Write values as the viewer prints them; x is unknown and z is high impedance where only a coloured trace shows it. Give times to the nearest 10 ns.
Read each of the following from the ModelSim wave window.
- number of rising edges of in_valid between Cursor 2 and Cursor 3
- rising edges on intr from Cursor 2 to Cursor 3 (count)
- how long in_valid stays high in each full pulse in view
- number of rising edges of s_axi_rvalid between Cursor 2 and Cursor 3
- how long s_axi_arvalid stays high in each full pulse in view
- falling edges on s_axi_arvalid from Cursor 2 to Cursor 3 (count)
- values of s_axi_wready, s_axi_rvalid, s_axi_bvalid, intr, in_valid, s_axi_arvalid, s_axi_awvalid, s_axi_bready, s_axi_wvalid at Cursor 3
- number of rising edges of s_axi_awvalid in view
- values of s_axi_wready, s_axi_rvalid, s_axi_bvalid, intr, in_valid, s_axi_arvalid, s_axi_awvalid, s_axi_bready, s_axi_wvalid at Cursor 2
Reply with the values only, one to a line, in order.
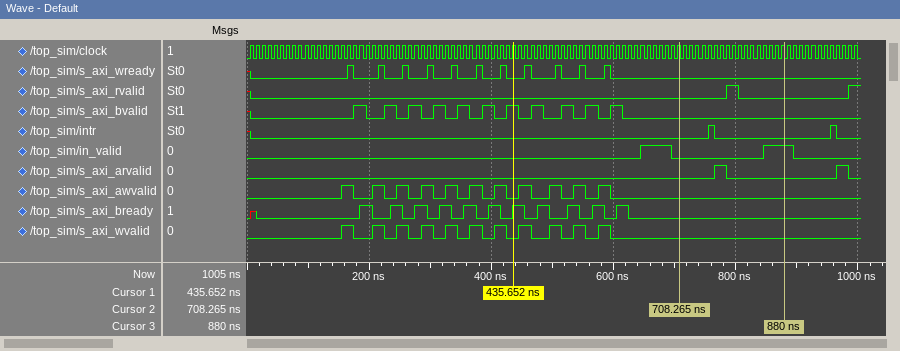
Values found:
1
1
50 ns, 50 ns
1
20 ns, 20 ns
1
s_axi_wready=0, s_axi_rvalid=0, s_axi_bvalid=0, intr=0, in_valid=1, s_axi_arvalid=0, s_axi_awvalid=0, s_axi_bready=0, s_axi_wvalid=0
11
s_axi_wready=0, s_axi_rvalid=0, s_axi_bvalid=0, intr=0, in_valid=0, s_axi_arvalid=0, s_axi_awvalid=0, s_axi_bready=0, s_axi_wvalid=0
